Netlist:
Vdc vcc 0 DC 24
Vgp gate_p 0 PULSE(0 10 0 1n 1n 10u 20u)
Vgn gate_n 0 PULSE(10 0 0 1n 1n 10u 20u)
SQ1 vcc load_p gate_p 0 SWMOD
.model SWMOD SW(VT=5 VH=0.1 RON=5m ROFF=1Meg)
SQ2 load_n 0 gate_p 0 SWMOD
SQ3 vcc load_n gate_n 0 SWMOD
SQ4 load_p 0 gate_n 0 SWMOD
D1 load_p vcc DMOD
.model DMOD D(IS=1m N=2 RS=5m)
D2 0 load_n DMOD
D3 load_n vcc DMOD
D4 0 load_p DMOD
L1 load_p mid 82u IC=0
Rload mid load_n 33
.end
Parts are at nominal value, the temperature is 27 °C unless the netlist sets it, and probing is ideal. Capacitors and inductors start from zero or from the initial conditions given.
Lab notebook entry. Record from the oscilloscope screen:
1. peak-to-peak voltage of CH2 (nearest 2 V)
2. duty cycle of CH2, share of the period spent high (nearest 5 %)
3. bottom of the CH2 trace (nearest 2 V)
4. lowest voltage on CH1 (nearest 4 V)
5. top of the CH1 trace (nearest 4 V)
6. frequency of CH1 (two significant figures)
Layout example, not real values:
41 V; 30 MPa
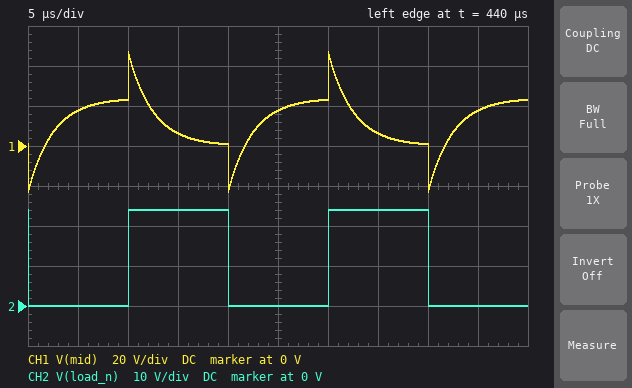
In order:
24 V; 50 %; 0 V; -24 V; 48 V; 50 kHz
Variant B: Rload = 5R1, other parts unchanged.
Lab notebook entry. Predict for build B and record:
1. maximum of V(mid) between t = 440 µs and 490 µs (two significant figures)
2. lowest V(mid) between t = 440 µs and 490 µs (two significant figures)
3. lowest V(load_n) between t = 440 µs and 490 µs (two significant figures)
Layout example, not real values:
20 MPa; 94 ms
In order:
31 V; -7.2 V; -7.1 mV
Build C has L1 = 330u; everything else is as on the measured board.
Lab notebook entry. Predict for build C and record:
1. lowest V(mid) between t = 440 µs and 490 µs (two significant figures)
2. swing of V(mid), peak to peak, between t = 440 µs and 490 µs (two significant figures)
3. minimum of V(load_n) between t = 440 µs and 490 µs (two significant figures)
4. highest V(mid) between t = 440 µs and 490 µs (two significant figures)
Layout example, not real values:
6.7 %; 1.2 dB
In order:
-11 V; 46 V; -1.7 mV; 35 V
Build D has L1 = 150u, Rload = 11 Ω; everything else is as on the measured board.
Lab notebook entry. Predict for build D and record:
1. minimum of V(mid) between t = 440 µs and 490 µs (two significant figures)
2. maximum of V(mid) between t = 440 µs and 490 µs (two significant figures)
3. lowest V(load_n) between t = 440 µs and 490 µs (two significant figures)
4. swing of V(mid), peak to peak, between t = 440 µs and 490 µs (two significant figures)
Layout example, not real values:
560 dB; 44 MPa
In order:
-8.4 V; 32 V; -3.8 mV; 41 V
